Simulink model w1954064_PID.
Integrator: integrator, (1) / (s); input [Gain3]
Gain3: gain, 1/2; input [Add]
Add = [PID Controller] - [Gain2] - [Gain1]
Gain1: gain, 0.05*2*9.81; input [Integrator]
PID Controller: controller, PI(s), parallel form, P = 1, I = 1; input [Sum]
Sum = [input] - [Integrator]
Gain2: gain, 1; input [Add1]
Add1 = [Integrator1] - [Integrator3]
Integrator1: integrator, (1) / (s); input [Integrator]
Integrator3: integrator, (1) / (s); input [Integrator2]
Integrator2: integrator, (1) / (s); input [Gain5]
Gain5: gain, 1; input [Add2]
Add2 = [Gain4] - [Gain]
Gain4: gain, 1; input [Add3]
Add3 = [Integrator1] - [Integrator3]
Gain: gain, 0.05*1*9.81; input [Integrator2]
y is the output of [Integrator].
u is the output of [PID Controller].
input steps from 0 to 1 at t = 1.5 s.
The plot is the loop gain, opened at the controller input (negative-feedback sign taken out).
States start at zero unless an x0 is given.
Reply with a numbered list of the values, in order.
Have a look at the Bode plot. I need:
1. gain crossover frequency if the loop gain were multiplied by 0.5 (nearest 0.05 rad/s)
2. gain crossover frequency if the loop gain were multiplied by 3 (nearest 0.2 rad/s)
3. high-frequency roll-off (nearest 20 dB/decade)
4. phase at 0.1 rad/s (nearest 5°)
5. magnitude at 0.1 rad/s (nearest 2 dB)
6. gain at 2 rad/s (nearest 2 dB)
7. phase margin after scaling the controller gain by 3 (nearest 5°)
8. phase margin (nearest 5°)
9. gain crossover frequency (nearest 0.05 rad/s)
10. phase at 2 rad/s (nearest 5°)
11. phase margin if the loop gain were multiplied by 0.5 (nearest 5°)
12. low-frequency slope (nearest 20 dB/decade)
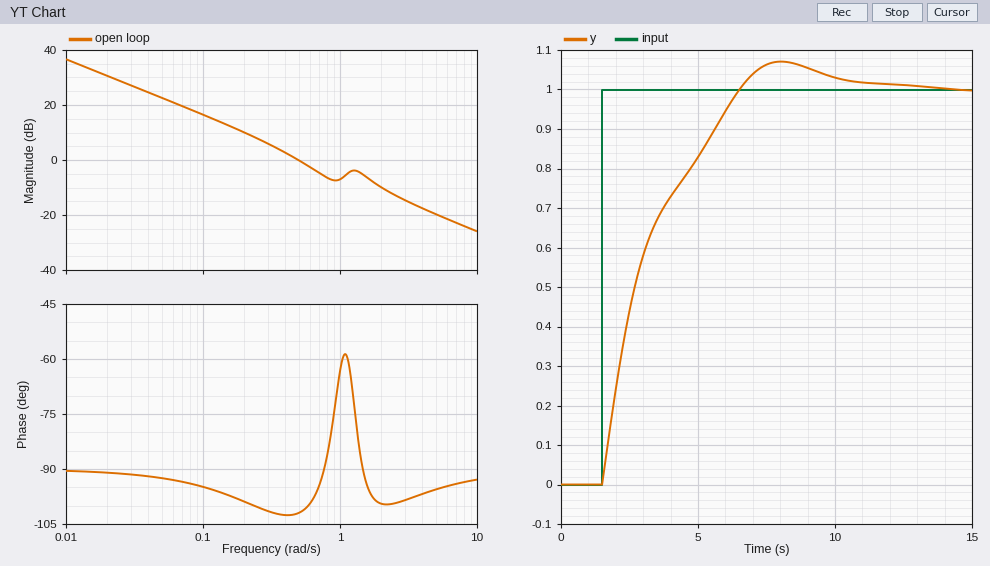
1. 0.30 rad/s
2. 2.0 rad/s
3. -20 dB/decade
4. -95°
5. 16 dB
6. -10 dB
7. 80°
8. 80°
9. 0.50 rad/s
10. -100°
11. 80°
12. -20 dB/decade
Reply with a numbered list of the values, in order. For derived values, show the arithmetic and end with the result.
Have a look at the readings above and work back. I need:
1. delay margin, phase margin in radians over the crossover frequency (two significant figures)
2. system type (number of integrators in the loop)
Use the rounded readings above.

1. 80 × π / 180 / 0.5 = 2.8 s
2. 1
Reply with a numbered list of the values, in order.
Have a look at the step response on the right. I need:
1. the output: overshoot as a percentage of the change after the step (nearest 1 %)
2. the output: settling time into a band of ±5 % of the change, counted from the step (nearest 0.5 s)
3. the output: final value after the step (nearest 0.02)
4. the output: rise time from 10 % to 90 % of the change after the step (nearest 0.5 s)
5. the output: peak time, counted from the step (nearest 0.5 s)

1. 7 %
2. 7.5 s
3. 1.00
4. 4.0 s
5. 6.5 s
